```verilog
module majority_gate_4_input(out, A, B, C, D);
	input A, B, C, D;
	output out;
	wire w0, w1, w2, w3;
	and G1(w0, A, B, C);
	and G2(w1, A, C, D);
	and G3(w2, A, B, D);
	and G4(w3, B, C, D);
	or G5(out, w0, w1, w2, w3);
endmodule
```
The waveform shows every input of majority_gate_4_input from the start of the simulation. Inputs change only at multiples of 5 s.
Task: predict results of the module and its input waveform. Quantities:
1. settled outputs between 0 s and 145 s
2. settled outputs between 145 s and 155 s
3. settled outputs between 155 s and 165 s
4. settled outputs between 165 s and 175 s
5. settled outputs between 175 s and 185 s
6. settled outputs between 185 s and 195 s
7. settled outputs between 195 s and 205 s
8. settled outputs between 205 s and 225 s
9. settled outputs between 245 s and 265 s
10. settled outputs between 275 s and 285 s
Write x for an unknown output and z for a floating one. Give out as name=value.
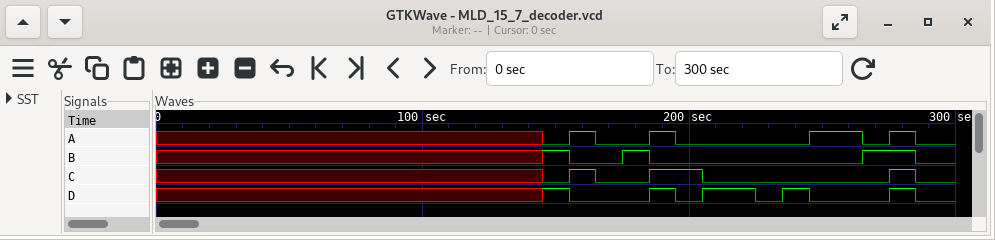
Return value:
out=x
out=0
out=0
out=0
out=0
out=1
out=0
out=0
out=0
out=1
